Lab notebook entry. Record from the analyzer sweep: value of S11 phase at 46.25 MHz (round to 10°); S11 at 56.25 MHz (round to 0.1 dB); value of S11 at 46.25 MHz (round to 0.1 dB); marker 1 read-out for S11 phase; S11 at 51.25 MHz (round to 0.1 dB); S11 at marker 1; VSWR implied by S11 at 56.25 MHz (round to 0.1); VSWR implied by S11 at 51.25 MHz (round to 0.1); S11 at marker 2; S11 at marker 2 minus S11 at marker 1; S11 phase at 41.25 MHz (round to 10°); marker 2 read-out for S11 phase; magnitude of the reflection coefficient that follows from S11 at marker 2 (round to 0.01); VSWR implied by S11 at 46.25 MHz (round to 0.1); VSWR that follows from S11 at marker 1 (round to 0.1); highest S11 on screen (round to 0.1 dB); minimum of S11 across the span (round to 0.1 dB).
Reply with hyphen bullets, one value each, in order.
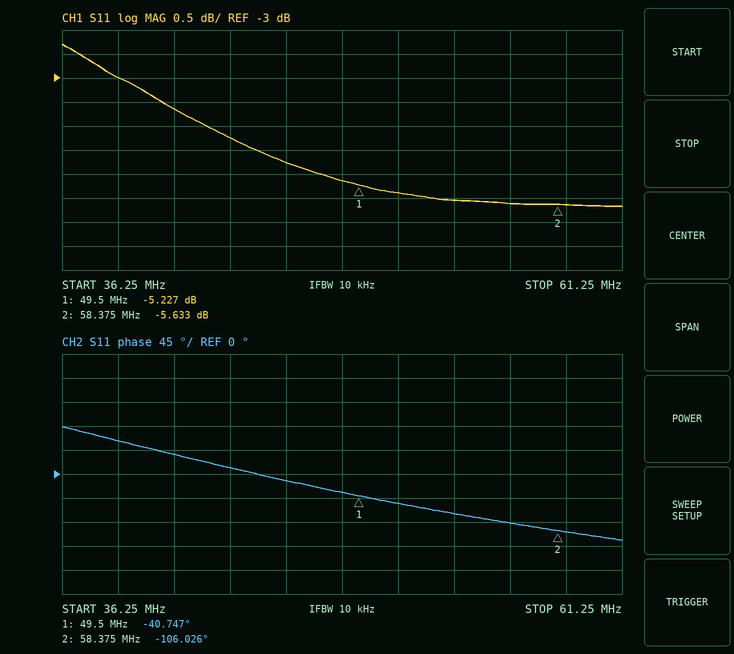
- -10°
- -5.6 dB
- -4.8 dB
- -40.747°
- -5.4 dB
- -5.227 dB
- 3.2
- 3.3
- -5.633 dB
- -0.406 dB
- 40°
- -106.026°
- 0.52
- 3.7
- 3.4
- -2.3 dB
- -5.7 dB
